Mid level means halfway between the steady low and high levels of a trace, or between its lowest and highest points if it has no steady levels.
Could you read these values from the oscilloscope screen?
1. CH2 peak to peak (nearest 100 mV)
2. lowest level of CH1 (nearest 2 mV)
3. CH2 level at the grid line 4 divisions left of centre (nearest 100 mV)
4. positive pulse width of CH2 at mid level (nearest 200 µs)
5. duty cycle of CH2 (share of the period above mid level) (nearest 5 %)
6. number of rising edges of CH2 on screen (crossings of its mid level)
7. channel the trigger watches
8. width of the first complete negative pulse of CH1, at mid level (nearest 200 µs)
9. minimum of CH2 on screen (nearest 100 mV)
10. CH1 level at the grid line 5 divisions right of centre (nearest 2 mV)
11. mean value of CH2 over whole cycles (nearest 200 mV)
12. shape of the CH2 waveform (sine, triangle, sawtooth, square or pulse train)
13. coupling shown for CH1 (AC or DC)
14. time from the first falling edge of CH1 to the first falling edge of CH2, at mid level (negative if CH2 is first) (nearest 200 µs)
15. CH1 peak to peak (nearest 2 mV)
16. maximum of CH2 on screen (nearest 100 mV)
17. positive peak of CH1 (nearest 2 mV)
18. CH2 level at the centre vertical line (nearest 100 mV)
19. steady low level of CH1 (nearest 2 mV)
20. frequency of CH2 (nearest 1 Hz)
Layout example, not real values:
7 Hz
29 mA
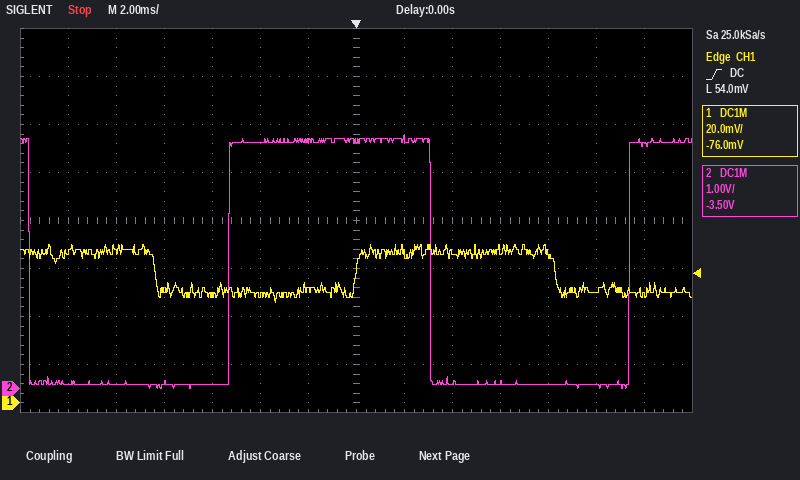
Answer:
5.3 V
42 mV
100 mV
8.4 ms
50 %
2
CH1
8.4 ms
0.0 V
46 mV
2.6 V
square
DC
-5.2 ms
24 mV
5.3 V
66 mV
5.2 V
46 mV
60 Hz
